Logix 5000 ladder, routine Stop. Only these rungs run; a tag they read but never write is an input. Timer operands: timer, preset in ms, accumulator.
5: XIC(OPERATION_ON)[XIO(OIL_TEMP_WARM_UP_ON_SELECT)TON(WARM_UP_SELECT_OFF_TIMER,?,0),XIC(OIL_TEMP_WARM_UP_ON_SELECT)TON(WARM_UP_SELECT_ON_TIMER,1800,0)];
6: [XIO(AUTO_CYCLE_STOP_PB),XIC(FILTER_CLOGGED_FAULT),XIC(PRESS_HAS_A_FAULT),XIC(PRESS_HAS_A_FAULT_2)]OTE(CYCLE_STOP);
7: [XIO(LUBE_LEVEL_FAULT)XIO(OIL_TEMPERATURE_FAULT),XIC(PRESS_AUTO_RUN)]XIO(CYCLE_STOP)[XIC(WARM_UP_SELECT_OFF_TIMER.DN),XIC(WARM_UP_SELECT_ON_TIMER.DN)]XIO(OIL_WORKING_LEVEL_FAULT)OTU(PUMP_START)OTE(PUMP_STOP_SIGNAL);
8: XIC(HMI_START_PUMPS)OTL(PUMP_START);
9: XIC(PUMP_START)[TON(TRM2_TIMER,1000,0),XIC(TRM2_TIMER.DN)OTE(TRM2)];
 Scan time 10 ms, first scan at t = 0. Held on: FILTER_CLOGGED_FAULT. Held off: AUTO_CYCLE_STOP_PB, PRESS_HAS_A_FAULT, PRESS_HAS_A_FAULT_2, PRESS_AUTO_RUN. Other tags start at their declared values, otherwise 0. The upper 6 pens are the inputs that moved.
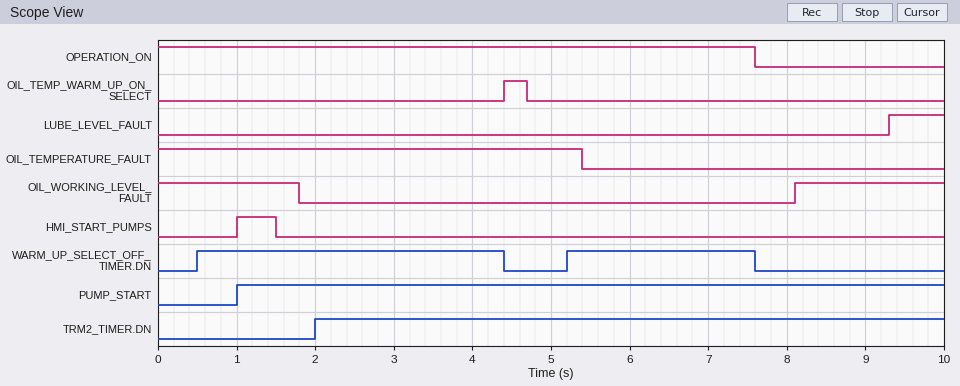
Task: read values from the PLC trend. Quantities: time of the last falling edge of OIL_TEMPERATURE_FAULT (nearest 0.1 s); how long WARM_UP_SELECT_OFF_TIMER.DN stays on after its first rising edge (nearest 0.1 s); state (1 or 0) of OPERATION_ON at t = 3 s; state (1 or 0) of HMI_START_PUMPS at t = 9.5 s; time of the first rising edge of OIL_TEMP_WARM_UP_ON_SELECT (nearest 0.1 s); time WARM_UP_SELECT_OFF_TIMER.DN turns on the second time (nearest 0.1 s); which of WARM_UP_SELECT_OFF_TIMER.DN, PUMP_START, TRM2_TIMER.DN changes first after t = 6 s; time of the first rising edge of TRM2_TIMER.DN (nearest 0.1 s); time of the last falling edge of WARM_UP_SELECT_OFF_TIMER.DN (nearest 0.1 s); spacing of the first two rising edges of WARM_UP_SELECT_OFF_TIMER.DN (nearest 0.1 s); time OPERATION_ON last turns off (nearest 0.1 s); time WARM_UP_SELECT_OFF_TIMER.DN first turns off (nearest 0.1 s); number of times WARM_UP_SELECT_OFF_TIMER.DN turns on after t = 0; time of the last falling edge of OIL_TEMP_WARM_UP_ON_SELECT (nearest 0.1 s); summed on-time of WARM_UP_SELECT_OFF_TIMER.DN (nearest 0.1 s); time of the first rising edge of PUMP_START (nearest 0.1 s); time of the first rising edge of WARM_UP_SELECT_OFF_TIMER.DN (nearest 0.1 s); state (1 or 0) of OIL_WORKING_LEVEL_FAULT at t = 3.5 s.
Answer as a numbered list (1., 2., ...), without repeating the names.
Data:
1. 5.4 s
2. 3.9 s
3. 1
4. 0
5. 4.4 s
6. 5.2 s
7. WARM_UP_SELECT_OFF_TIMER.DN
8. 2.0 s
9. 7.6 s
10. 4.7 s
11. 7.6 s
12. 4.4 s
13. 2
14. 4.7 s
15. 6.3 s
16. 1.0 s
17. 0.5 s
18. 0
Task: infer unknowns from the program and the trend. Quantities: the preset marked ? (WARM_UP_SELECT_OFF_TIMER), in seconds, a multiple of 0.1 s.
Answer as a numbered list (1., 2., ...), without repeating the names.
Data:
1. 0.5 s
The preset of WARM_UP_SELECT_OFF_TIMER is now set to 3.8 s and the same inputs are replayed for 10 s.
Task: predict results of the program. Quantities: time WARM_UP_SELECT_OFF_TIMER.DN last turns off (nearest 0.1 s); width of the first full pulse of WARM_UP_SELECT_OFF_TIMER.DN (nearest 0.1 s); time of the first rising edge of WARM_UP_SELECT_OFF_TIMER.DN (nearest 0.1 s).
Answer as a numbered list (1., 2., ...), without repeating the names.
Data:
1. 4.4 s
2. 0.6 s
3. 3.8 s
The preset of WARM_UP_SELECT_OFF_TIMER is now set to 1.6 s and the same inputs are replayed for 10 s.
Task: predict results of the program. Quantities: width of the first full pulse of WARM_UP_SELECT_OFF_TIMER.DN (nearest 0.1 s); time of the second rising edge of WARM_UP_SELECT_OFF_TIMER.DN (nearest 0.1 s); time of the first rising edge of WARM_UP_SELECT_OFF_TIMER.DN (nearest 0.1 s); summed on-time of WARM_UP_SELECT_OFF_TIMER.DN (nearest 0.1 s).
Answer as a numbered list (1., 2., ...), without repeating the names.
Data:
1. 2.8 s
2. 6.3 s
3. 1.6 s
4. 4.1 s
